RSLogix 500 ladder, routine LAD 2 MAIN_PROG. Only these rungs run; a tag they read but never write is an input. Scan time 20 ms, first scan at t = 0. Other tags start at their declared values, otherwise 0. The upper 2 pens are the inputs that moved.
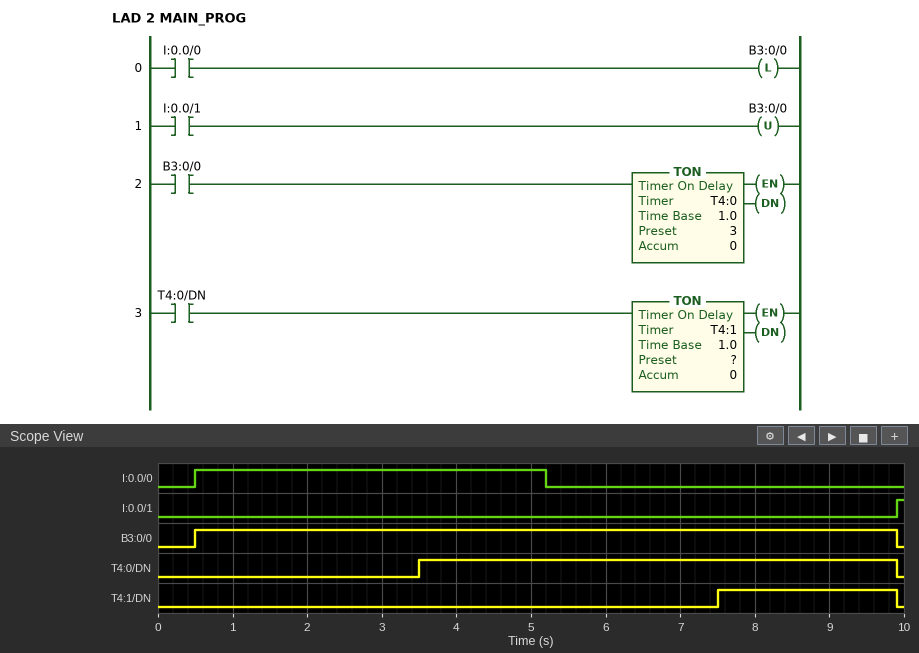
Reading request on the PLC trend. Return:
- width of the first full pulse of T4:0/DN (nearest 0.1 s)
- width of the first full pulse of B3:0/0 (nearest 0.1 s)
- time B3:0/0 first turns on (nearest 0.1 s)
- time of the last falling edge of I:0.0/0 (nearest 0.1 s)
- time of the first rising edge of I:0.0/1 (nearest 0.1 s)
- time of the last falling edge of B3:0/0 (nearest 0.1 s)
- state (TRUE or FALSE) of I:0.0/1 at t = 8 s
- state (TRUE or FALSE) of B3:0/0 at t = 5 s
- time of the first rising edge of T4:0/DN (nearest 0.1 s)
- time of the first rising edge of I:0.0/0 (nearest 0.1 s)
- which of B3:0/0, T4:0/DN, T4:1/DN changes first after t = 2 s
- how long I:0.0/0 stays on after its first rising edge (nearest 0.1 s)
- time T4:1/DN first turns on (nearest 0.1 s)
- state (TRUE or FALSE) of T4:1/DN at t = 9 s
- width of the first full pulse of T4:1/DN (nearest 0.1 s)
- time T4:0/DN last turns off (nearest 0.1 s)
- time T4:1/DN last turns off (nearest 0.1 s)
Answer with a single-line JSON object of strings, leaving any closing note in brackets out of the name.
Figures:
{"width of the first full pulse of T4:0/DN": "6.4 s", "width of the first full pulse of B3:0/0": "9.4 s", "time B3:0/0 first turns on": "0.5 s", "time of the last falling edge of I:0.0/0": "5.2 s", "time of the first rising edge of I:0.0/1": "9.9 s", "time of the last falling edge of B3:0/0": "9.9 s", "state (TRUE or FALSE) of I:0.0/1 at t = 8 s": "FALSE", "state (TRUE or FALSE) of B3:0/0 at t = 5 s": "TRUE", "time of the first rising edge of T4:0/DN": "3.5 s", "time of the first rising edge of I:0.0/0": "0.5 s", "which of B3:0/0, T4:0/DN, T4:1/DN changes first after t = 2 s": "T4:0/DN", "how long I:0.0/0 stays on after its first rising edge": "4.7 s", "time T4:1/DN first turns on": "7.5 s", "state (TRUE or FALSE) of T4:1/DN at t = 9 s": "TRUE", "width of the first full pulse of T4:1/DN": "2.4 s", "time T4:0/DN last turns off": "9.9 s", "time T4:1/DN last turns off": "9.9 s"}
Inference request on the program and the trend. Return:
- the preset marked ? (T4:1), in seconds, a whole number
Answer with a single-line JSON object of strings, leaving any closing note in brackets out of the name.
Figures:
{"the preset marked ? (T4:1), in seconds, a whole number": "4 s"}
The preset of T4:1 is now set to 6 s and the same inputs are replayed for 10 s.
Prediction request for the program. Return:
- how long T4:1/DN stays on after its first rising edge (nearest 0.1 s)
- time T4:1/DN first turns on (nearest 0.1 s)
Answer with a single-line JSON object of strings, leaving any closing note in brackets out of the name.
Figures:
{"how long T4:1/DN stays on after its first rising edge": "0.4 s", "time T4:1/DN first turns on": "9.5 s"}
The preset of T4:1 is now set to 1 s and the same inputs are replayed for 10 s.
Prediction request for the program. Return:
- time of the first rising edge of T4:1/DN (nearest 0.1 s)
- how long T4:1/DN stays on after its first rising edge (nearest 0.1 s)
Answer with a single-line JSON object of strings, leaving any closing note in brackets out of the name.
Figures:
{"time of the first rising edge of T4:1/DN": "4.5 s", "how long T4:1/DN stays on after its first rising edge": "5.4 s"}
